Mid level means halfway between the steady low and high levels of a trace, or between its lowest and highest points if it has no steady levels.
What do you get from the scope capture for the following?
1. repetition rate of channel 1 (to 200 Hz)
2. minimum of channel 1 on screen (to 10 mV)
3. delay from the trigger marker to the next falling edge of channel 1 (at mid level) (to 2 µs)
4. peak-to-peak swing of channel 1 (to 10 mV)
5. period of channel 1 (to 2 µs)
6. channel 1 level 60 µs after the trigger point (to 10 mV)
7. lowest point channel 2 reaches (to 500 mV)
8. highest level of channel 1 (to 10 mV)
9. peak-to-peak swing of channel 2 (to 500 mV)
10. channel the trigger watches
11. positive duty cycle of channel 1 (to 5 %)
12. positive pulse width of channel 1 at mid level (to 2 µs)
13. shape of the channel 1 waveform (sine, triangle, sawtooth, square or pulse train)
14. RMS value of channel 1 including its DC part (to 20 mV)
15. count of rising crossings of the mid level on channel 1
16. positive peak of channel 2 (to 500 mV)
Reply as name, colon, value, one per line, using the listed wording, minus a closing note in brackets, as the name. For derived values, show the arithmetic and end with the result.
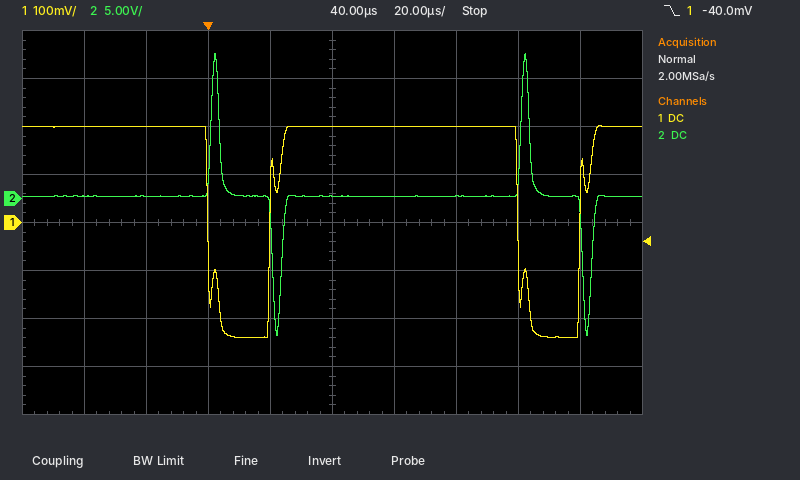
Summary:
repetition rate of channel 1: 1 / 100 µs ≈ 10.0 kHz
minimum of channel 1 on screen: -240 mV
delay from the trigger marker to the next falling edge of channel 1 (at mid level): 100 µs
peak-to-peak swing of channel 1: 200 mV − (-240 mV) = 440 mV
period of channel 1: 100 µs
channel 1 level 60 µs after the trigger point: 200 mV
lowest point channel 2 reaches: -14.5 V
highest level of channel 1: 200 mV
peak-to-peak swing of channel 2: 15.0 V − (-14.5 V) = 29.5 V
channel the trigger watches: channel 1
positive duty cycle of channel 1: 80 µs / 100 µs ≈ 80 %
positive pulse width of channel 1 at mid level: 80 µs
shape of the channel 1 waveform: pulse train
RMS value of channel 1 including its DC part: √(0.8 × (200 mV)² + 0.2 × (-240 mV)²) ≈ 209 mV, so 200 mV to the nearest 20 mV
count of rising crossings of the mid level on channel 1: 2
positive peak of channel 2: 15.0 V
